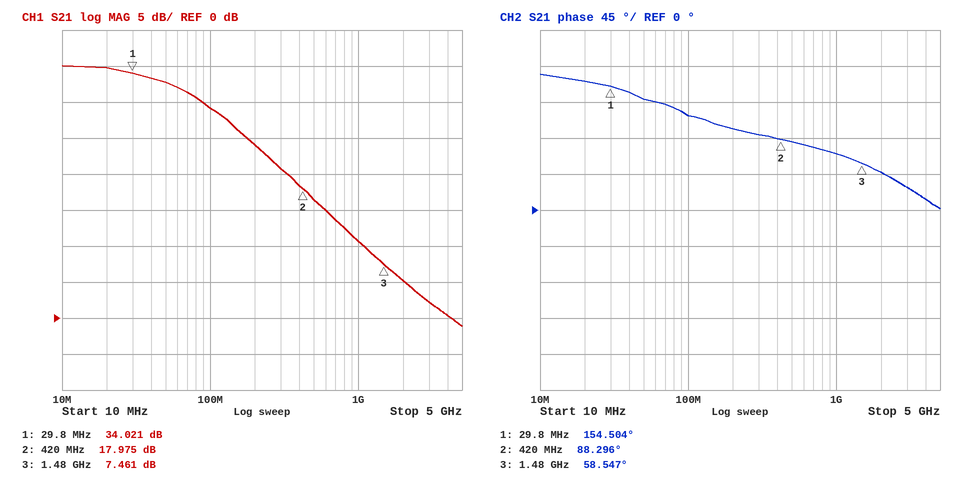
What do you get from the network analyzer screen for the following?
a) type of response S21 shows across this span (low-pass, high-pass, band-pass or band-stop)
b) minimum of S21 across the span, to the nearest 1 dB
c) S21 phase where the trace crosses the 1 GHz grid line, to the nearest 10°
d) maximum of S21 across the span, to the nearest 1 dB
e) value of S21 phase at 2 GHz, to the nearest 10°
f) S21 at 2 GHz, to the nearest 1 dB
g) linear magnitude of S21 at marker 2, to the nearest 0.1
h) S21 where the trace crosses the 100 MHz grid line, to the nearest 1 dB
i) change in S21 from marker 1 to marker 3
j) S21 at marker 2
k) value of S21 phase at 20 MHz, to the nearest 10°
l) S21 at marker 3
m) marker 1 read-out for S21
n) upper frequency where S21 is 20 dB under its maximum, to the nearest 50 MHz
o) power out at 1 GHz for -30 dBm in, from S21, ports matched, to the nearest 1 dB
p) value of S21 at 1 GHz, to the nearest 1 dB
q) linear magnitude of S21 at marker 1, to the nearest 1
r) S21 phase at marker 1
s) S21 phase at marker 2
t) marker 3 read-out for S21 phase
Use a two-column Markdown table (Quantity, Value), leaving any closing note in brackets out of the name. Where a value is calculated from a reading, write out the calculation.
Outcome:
| Quantity | Value |
|---|---|
| type of response S21 shows across this span | low-pass |
| minimum of S21 across the span, to the nearest 1 dB | -1 dB |
| S21 phase where the trace crosses the 1 GHz grid line, to the nearest 10° | 70° |
| maximum of S21 across the span, to the nearest 1 dB | 35 dB |
| value of S21 phase at 2 GHz, to the nearest 10° | 50° |
| S21 at 2 GHz, to the nearest 1 dB | 5 dB |
| linear magnitude of S21 at marker 2, to the nearest 0.1 | 10^(17.975/20) ≈ 7.9 |
| S21 where the trace crosses the 100 MHz grid line, to the nearest 1 dB | 29 dB |
| change in S21 from marker 1 to marker 3 | 7.461 − (34.021) = -26.560 dB |
| S21 at marker 2 | 17.975 dB |
| value of S21 phase at 20 MHz, to the nearest 10° | 160° |
| S21 at marker 3 | 7.461 dB |
| marker 1 read-out for S21 | 34.021 dB |
| upper frequency where S21 is 20 dB under its maximum, to the nearest 50 MHz | 600 MHz |
| power out at 1 GHz for -30 dBm in, from S21, ports matched, to the nearest 1 dB | -30 dBm + (11 dB) = -19 dBm |
| value of S21 at 1 GHz, to the nearest 1 dB | 11 dB |
| linear magnitude of S21 at marker 1, to the nearest 1 | 10^(34.021/20) ≈ 50 |
| S21 phase at marker 1 | 154.504° |
| S21 phase at marker 2 | 88.296° |
| marker 3 read-out for S21 phase | 58.547° |
